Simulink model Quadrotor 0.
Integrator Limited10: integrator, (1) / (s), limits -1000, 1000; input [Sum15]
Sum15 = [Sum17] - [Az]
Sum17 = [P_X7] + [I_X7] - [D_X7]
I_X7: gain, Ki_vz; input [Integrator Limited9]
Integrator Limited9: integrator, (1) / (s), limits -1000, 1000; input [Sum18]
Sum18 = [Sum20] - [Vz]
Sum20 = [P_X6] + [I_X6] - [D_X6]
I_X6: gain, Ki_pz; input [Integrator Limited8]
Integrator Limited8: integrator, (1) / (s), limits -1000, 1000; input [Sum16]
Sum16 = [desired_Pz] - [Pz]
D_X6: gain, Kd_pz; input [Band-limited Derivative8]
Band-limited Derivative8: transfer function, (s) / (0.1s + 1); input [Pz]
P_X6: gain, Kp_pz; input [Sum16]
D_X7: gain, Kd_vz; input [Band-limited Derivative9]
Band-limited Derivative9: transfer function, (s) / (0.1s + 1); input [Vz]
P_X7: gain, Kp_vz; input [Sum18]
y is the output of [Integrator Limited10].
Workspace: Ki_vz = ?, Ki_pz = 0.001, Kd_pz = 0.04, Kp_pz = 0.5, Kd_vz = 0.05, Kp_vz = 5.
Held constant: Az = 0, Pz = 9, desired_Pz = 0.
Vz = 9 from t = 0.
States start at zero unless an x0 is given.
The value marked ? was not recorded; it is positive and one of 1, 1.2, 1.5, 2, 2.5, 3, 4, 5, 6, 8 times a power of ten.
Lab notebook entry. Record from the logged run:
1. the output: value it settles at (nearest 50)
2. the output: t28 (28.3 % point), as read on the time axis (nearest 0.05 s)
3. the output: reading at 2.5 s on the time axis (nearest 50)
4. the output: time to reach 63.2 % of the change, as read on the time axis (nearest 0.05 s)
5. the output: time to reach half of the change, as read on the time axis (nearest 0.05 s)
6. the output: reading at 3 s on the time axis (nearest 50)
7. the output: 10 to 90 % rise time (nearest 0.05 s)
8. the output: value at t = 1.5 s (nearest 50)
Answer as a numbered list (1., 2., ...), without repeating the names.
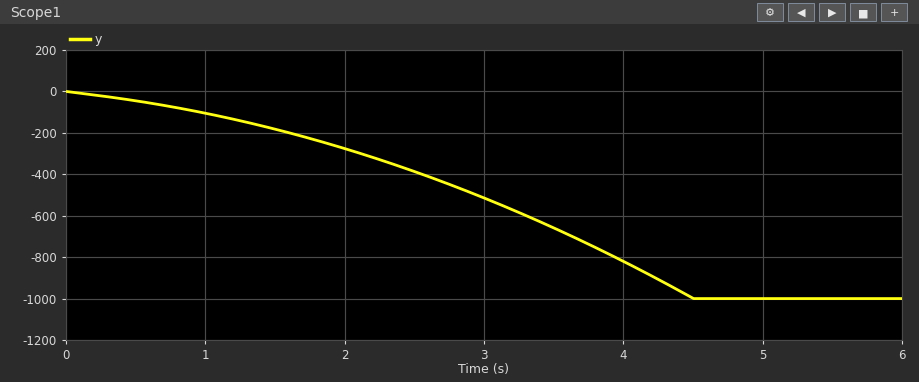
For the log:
1. -1000
2. 2.05 s
3. -400
4. 3.40 s
5. 2.95 s
6. -500
7. 3.25 s
8. -200
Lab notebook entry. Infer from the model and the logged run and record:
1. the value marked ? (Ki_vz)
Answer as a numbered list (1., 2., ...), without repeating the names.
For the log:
1. 5
